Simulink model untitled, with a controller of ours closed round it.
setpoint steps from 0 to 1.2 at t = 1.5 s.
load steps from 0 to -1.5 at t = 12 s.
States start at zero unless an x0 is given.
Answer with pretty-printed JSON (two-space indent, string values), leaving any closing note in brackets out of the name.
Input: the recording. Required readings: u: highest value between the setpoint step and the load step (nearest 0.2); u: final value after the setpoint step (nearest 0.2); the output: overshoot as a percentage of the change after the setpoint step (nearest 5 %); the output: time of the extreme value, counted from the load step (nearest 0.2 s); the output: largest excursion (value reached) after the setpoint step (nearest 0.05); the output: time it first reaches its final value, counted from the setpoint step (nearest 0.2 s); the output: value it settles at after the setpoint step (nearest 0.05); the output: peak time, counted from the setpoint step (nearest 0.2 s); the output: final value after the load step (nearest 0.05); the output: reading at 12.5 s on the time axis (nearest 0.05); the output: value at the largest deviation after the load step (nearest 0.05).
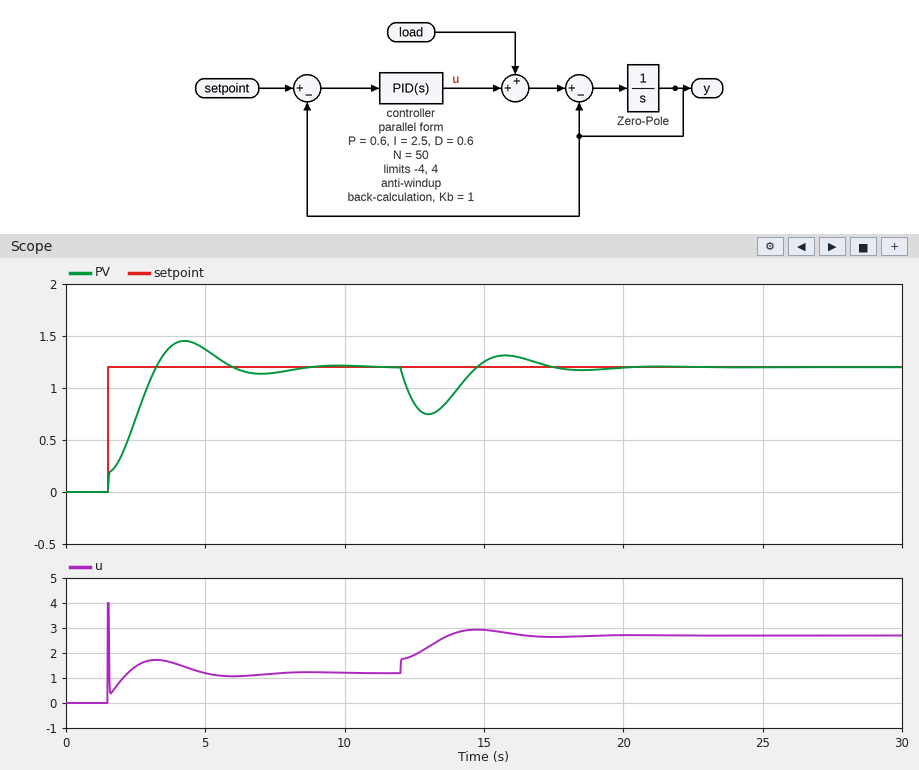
{
  "u: highest value between the setpoint step and the load step": "4.0",
  "u: final value after the setpoint step": "1.2",
  "the output: overshoot as a percentage of the change after the setpoint step": "20 %",
  "the output: time of the extreme value, counted from the load step": "1.0 s",
  "the output: largest excursion (value reached) after the setpoint step": "1.45",
  "the output: time it first reaches its final value, counted from the setpoint step": "1.8 s",
  "the output: value it settles at after the setpoint step": "1.20",
  "the output: peak time, counted from the setpoint step": "2.8 s",
  "the output: final value after the load step": "1.20",
  "the output: reading at 12.5 s on the time axis": "0.85",
  "the output: value at the largest deviation after the load step": "0.75"
}
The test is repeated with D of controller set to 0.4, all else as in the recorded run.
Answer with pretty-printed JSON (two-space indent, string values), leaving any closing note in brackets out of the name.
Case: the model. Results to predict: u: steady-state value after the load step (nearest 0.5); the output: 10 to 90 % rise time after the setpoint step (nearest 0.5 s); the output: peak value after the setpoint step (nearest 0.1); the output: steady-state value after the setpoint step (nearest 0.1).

{
  "u: steady-state value after the load step": "2.5",
  "the output: 10 to 90 % rise time after the setpoint step": "1.5 s",
  "the output: peak value after the setpoint step": "1.4",
  "the output: steady-state value after the setpoint step": "1.2"
}
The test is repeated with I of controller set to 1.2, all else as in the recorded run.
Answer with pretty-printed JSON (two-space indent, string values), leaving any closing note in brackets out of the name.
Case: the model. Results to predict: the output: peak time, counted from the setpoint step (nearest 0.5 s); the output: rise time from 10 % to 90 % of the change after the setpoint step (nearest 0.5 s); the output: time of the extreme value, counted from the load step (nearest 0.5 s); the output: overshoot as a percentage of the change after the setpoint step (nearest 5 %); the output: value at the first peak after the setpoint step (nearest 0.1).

{
  "the output: peak time, counted from the setpoint step": "4.5 s",
  "the output: rise time from 10 % to 90 % of the change after the setpoint step": "2.5 s",
  "the output: time of the extreme value, counted from the load step": "1.5 s",
  "the output: overshoot as a percentage of the change after the setpoint step": "10 %",
  "the output: value at the first peak after the setpoint step": "1.3"
}
